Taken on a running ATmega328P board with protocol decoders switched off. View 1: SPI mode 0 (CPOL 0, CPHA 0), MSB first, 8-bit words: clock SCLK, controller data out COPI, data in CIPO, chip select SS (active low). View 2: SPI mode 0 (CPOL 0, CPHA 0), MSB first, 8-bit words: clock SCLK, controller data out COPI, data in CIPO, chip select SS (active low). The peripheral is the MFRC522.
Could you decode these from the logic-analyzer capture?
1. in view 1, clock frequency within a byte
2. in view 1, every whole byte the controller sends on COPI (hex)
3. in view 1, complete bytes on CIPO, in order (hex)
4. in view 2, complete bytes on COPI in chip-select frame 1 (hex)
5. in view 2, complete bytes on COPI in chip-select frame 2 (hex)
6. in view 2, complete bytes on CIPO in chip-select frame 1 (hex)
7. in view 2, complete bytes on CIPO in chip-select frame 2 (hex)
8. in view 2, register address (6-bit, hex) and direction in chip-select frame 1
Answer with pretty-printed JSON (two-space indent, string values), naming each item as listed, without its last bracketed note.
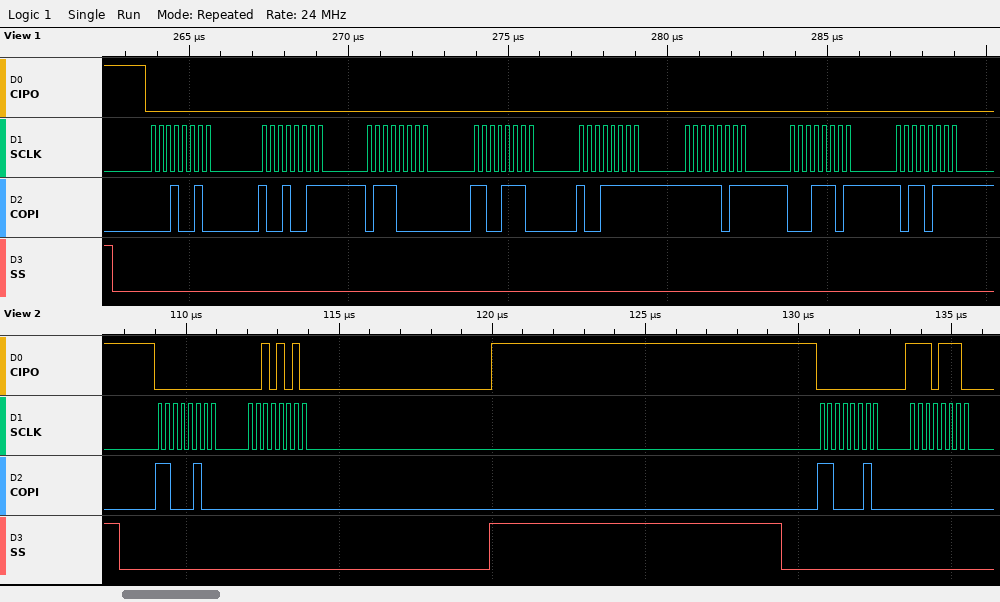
{
  "in view 1, clock frequency within a byte": "4 MHz",
  "in view 1, every whole byte the controller sends on COPI": "12 93 70 CE 9F FB 1D B7",
  "in view 1, complete bytes on CIPO, in order": "00 00 00 00 00 00 00 00",
  "in view 2, complete bytes on COPI in chip-select frame 1": "C4 00",
  "in view 2, complete bytes on COPI in chip-select frame 2": "C2 00",
  "in view 2, complete bytes on CIPO in chip-select frame 1": "00 2A",
  "in view 2, complete bytes on CIPO in chip-select frame 2": "00 EE",
  "in view 2, register address (6-bit, hex) and direction in chip-select frame 1": "0x22 read"
}
